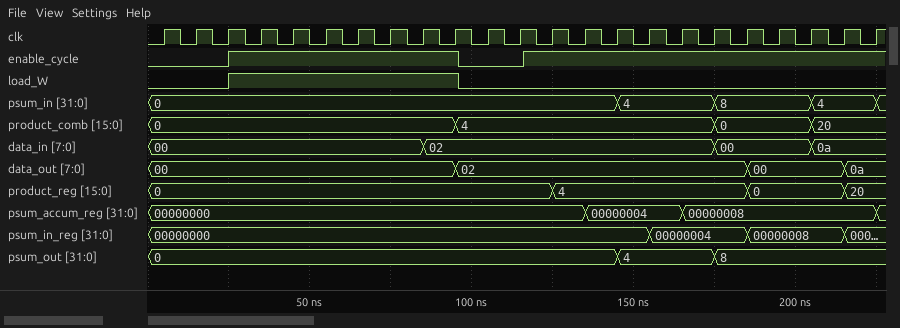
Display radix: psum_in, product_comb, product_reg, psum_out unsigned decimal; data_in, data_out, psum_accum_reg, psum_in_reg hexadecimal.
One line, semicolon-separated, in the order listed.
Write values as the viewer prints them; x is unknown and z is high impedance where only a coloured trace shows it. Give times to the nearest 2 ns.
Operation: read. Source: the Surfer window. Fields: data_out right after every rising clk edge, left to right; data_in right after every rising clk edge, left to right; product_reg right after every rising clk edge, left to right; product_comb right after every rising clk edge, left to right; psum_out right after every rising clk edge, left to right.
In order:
00, 00, 00, 00, 00, 00, 00, 00, 00, 02, 02, 02, 02, 02, 02, 02, 02, 02, 00, 00, 00, 0a, 0a; 00, 00, 00, 00, 00, 00, 00, 00, 02, 02, 02, 02, 02, 02, 02, 02, 02, 00, 00, 00, 0a, 0a, 0a; 0, 0, 0, 0, 0, 0, 0, 0, 0, 0, 0, 0, 4, 4, 4, 4, 4, 4, 0, 0, 0, 20, 20; 0, 0, 0, 0, 0, 0, 0, 0, 0, 4, 4, 4, 4, 4, 4, 4, 4, 0, 0, 0, 20, 20, 20; 0, 0, 0, 0, 0, 0, 0, 0, 0, 0, 0, 0, 0, 0, 4, 4, 4, 8, 8, 8, 8, 8, 8
